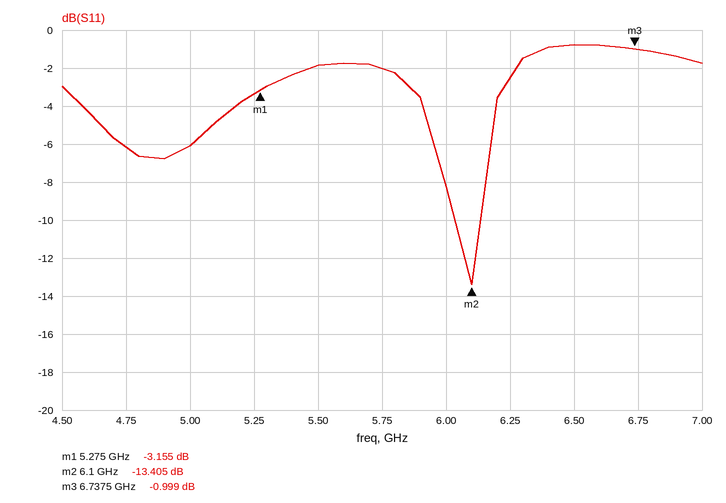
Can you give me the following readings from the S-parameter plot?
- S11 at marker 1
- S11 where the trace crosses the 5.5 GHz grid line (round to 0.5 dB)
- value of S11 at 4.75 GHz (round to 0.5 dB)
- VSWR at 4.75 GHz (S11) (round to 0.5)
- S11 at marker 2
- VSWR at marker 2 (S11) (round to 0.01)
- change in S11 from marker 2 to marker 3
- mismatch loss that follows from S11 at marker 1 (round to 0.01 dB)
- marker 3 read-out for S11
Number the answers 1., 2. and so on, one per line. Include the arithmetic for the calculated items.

1. -3.155 dB
2. -2.0 dB
3. -6.0 dB
4. |Γ| = 10^(-6/20) = 0.5012; VSWR = (1 + 0.5012)/(1 − 0.5012) ≈ 3.0
5. -13.405 dB
6. (1 + 0.2137)/(1 − 0.2137) ≈ 1.54
7. -0.999 − (-13.405) = 12.406 dB
8. −10 log10(1 − 10^(-3.155/10)) ≈ 2.87 dB
9. -0.999 dB
